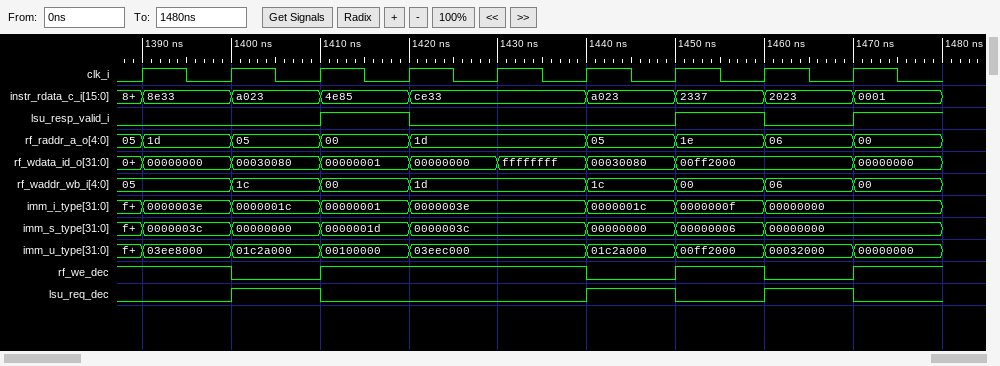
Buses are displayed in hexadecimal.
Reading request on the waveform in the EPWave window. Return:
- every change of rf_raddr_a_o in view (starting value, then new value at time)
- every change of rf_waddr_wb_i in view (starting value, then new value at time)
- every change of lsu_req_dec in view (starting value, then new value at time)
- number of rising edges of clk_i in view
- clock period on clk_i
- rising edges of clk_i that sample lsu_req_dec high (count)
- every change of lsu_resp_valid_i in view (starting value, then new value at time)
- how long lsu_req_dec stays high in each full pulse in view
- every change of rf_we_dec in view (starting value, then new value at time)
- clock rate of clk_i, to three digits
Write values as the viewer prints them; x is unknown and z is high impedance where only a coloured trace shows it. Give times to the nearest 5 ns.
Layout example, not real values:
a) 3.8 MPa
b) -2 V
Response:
a) 05, 1d at 1390 ns, 05 at 1400 ns, 00 at 1410 ns, 1d at 1420 ns, 05 at 1440 ns, 1e at 1450 ns, 06 at 1460 ns, 00 at 1470 ns
b) 05, 1c at 1400 ns, 00 at 1410 ns, 1d at 1420 ns, 1c at 1440 ns, 00 at 1450 ns, 06 at 1460 ns, 00 at 1470 ns
c) 0, 1 at 1400 ns, 0 at 1410 ns, 1 at 1440 ns, 0 at 1450 ns, 1 at 1460 ns, 0 at 1470 ns
d) 9
e) 10 ns
f) 3
g) 0, 1 at 1410 ns, 0 at 1420 ns, 1 at 1450 ns, 0 at 1460 ns, 1 at 1470 ns
h) 10 ns, 10 ns, 10 ns
i) 1, 0 at 1400 ns, 1 at 1410 ns, 0 at 1440 ns, 1 at 1450 ns, 0 at 1460 ns, 1 at 1470 ns
j) 100 MHz
